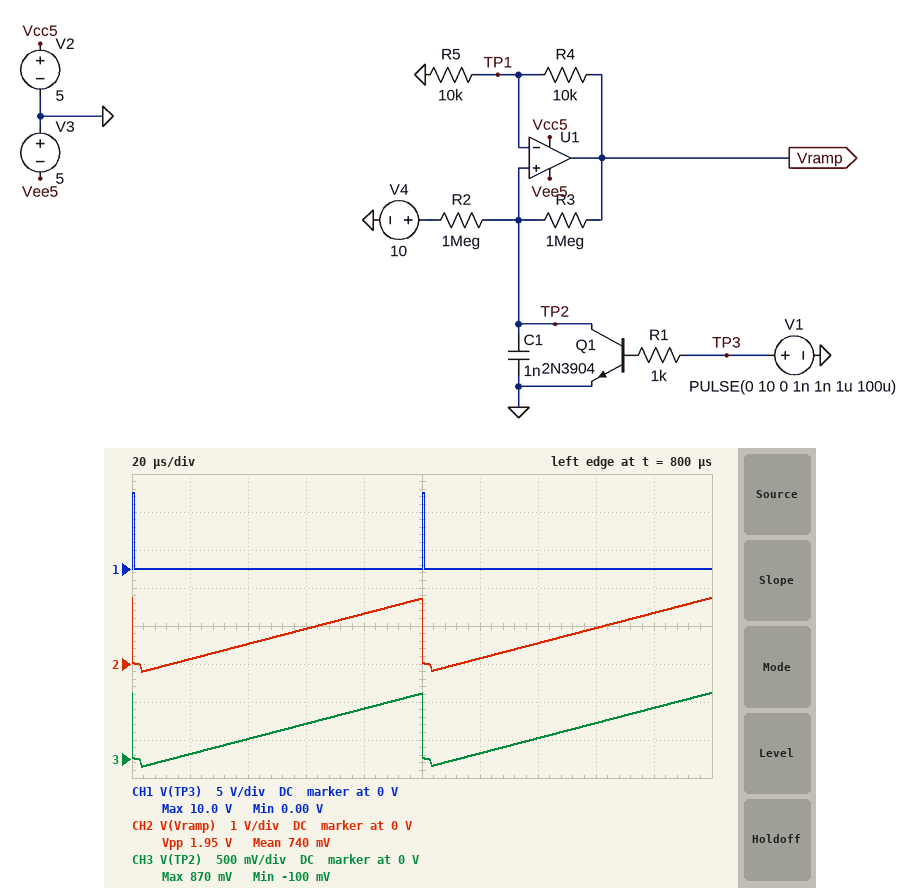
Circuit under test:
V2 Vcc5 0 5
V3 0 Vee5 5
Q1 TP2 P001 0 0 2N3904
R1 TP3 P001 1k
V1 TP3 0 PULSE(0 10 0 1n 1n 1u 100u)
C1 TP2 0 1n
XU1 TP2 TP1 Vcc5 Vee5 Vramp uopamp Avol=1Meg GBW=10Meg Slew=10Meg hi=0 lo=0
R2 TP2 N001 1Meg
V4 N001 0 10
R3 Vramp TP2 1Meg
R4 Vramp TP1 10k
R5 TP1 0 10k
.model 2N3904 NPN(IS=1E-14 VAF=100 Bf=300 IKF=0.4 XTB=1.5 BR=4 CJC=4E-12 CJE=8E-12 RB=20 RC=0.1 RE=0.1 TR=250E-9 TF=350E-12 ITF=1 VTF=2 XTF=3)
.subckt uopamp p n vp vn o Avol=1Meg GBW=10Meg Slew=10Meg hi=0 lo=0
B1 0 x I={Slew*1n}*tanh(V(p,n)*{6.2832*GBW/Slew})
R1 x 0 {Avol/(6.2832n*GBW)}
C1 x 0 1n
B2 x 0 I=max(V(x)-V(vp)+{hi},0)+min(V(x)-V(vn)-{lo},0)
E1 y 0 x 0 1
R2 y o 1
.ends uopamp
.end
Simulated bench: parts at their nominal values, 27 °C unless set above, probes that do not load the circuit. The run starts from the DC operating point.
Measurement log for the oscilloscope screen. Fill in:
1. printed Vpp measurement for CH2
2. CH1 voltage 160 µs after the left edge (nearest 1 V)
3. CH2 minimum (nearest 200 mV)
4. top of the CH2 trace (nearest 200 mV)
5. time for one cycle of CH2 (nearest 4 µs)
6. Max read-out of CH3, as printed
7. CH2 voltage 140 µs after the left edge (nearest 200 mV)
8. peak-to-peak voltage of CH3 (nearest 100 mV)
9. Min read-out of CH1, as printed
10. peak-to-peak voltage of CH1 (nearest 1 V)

1.95 V
0 V
-200 mV
1.8 V
100 µs
870 mV
600 mV
1.0 V
0.00 V
10 V
